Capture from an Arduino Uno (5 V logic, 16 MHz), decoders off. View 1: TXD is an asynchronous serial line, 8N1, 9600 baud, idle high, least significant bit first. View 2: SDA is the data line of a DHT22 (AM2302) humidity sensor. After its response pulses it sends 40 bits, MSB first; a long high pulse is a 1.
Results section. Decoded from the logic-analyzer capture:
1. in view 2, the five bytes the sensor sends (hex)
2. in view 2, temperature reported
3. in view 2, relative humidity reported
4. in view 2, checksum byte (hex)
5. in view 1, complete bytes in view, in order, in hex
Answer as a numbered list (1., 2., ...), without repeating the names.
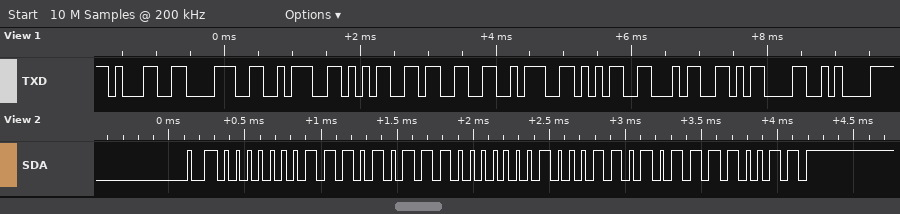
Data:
1. 01 D7 01 1A F3
2. 28.2 °C
3. 47.1 %
4. 0xF3
5. 0x31 0x38 0x3A 0x35 0x33 0x3A 0x35 0x34 0x0D 0x0A
